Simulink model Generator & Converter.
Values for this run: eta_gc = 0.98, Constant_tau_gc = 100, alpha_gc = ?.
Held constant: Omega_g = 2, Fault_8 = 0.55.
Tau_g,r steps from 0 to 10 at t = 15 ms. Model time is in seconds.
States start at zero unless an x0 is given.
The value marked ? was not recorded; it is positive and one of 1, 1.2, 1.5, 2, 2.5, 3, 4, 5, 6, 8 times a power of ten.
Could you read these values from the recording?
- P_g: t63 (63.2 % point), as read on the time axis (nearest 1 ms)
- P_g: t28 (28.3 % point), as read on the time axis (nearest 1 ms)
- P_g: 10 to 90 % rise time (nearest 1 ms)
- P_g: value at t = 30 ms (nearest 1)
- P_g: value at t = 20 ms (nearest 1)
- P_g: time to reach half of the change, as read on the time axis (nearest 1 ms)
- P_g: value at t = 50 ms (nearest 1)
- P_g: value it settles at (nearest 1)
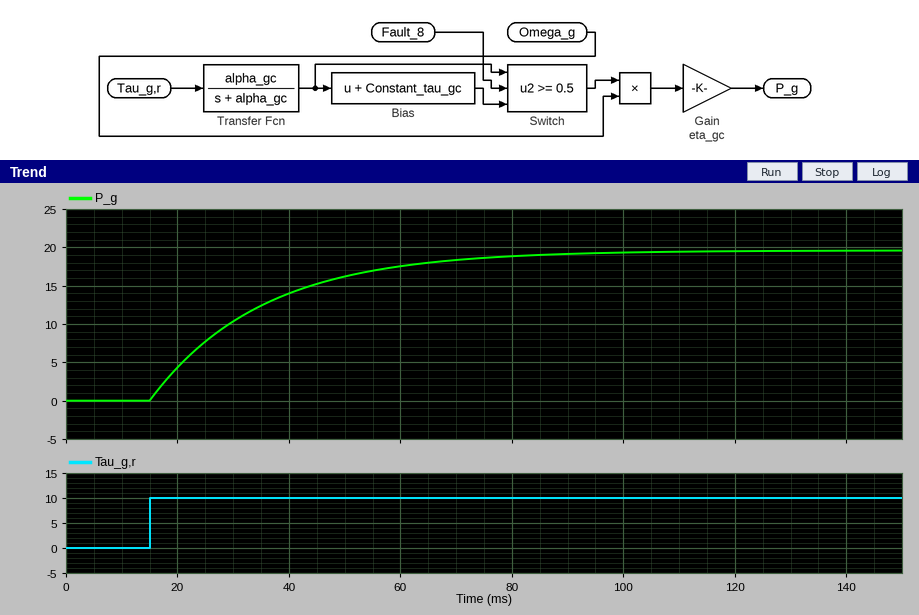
35 ms
22 ms
44 ms
10
4
29 ms
16
20
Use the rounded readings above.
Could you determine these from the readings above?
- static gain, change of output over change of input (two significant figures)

2.0
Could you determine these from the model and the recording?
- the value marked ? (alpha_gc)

50
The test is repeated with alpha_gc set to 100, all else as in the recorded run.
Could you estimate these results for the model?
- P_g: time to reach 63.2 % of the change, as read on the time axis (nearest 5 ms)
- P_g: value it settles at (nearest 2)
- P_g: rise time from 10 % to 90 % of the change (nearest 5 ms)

25 ms
20
20 ms
